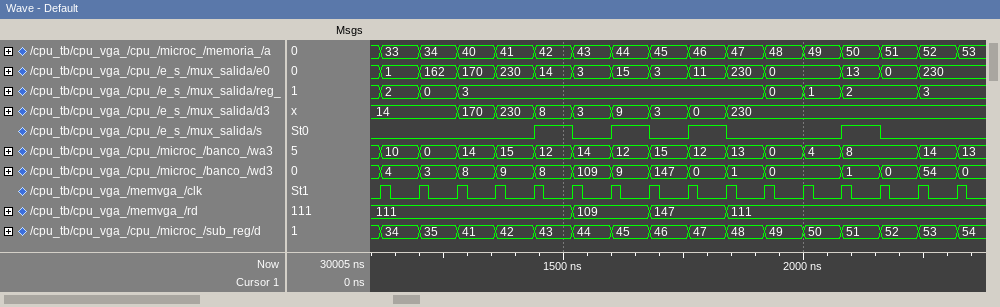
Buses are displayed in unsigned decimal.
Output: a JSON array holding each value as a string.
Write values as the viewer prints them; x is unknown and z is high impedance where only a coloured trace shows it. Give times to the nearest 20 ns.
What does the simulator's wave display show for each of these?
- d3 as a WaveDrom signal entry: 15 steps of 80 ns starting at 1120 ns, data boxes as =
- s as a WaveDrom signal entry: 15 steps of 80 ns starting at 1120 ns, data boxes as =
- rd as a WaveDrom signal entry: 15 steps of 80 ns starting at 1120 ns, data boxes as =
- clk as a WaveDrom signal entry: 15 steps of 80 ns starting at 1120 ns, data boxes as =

["{name: 'd3', wave: '=.========.....', data: '14 170 230 8 3 9 3 0 230'}", "{name: 's', wave: '0...101010..10.'}", "{name: 'rd', wave: '=....=.=.=.....', data: '111 109 147 111'}", "{name: 'clk', wave: 'p..............'}"]
